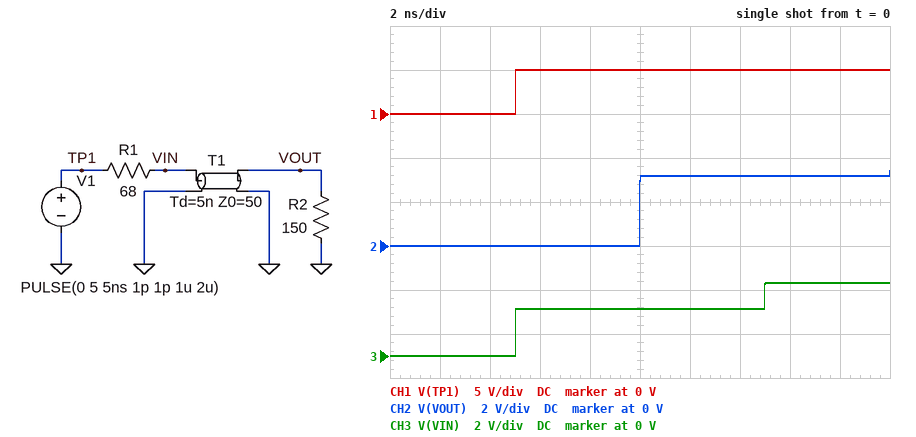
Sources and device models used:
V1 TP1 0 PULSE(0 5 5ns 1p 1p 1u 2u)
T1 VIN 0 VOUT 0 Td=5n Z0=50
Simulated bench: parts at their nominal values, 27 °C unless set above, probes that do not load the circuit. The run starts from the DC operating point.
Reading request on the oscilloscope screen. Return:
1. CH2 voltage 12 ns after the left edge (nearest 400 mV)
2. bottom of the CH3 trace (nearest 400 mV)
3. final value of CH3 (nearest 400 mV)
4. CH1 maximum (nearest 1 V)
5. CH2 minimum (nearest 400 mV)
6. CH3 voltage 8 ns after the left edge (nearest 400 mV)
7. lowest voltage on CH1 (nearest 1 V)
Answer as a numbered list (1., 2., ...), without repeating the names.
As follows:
1. 3.2 V
2. 0 V
3. 3.2 V
4. 5 V
5. 0 V
6. 2.0 V
7. 0 V
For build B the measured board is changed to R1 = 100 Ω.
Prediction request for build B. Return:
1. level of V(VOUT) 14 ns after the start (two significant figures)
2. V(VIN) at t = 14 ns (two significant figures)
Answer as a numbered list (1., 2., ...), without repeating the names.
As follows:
1. 2.5 V
2. 1.7 V
